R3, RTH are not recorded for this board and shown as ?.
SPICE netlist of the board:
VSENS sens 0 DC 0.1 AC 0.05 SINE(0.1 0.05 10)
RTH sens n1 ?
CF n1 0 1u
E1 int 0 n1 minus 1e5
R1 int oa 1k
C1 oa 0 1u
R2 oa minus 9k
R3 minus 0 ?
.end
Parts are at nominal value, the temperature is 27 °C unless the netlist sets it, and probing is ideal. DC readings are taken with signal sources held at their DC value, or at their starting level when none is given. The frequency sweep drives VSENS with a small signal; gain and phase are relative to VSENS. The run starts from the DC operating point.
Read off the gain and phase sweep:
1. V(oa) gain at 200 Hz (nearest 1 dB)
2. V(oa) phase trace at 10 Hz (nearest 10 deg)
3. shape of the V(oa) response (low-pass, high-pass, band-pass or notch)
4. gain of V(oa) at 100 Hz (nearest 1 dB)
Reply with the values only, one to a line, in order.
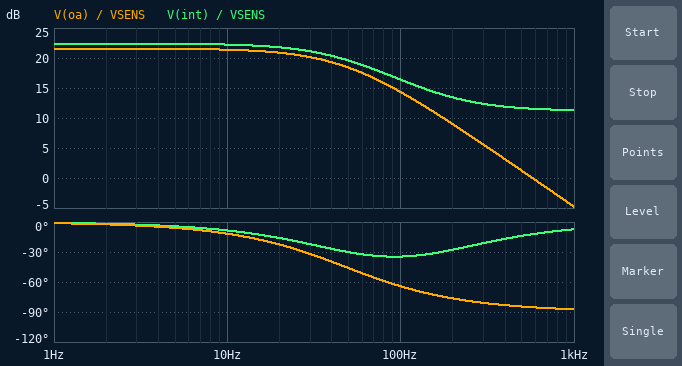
9 dB
-10 deg
low-pass
14 dB
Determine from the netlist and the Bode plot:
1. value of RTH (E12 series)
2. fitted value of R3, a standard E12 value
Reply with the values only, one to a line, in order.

3.3 kΩ
820 Ω
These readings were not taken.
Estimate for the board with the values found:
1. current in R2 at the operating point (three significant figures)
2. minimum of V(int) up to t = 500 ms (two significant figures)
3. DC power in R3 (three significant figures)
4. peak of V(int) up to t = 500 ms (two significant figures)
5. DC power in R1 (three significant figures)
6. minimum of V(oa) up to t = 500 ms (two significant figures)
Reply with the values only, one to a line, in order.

122 µA
670 mV
12.2 µW
2.0 V
14.9 µW
610 mV
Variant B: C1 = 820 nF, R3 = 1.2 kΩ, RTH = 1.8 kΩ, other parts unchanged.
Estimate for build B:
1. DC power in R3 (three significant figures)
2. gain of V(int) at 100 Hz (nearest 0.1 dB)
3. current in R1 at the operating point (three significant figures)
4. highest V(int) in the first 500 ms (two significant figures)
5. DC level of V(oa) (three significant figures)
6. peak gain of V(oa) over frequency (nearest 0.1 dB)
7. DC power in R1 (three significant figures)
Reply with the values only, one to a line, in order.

8.33 µW
16.7 dB
83.3 µA
1.4 V
850 mV
18.6 dB
6.94 µW
